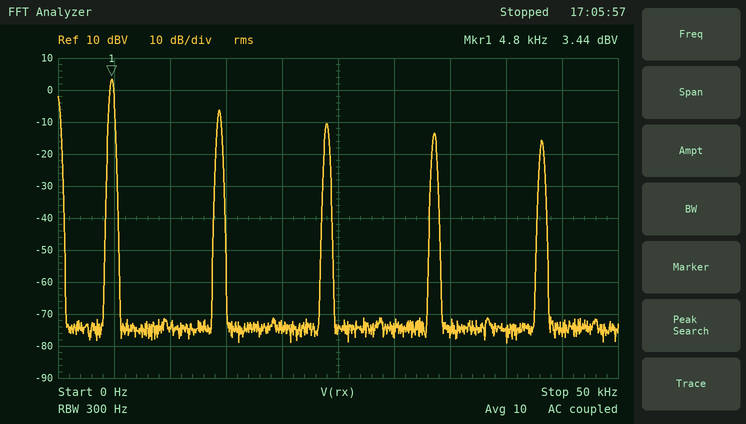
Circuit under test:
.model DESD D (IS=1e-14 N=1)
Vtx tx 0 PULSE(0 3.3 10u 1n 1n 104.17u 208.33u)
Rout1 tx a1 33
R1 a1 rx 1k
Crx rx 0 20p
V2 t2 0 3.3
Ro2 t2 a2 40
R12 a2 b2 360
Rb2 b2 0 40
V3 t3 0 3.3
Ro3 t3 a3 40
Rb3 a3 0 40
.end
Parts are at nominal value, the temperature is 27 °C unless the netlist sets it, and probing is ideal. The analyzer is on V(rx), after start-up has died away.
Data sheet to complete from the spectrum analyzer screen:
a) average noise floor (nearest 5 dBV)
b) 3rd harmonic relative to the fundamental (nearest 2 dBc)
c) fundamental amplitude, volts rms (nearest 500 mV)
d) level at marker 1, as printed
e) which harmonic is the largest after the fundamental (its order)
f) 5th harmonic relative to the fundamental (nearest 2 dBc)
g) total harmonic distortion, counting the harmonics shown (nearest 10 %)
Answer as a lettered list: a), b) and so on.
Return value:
a) -75 dBV
b) -10 dBc
c) 1.5 V
d) 3.44 dBV
e) 3
f) -14 dBc
g) 40 %
